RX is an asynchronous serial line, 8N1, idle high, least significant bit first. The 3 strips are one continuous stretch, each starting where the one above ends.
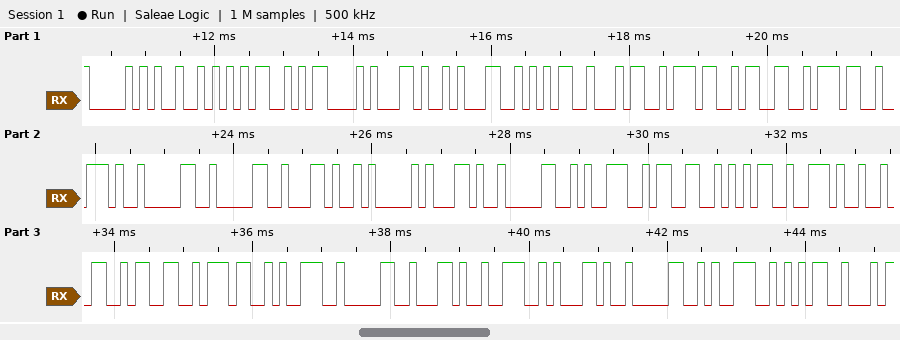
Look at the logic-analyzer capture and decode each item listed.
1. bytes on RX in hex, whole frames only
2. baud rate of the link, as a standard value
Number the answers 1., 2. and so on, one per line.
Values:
1. 50 52 4D 43 2C 31 35 34 37 33 37 2E 30 30 2C 41 2C 30 39 33 35 2E 32 33 37 39 30 2C 4E 2C 30 39 35
2. 9600 baud
